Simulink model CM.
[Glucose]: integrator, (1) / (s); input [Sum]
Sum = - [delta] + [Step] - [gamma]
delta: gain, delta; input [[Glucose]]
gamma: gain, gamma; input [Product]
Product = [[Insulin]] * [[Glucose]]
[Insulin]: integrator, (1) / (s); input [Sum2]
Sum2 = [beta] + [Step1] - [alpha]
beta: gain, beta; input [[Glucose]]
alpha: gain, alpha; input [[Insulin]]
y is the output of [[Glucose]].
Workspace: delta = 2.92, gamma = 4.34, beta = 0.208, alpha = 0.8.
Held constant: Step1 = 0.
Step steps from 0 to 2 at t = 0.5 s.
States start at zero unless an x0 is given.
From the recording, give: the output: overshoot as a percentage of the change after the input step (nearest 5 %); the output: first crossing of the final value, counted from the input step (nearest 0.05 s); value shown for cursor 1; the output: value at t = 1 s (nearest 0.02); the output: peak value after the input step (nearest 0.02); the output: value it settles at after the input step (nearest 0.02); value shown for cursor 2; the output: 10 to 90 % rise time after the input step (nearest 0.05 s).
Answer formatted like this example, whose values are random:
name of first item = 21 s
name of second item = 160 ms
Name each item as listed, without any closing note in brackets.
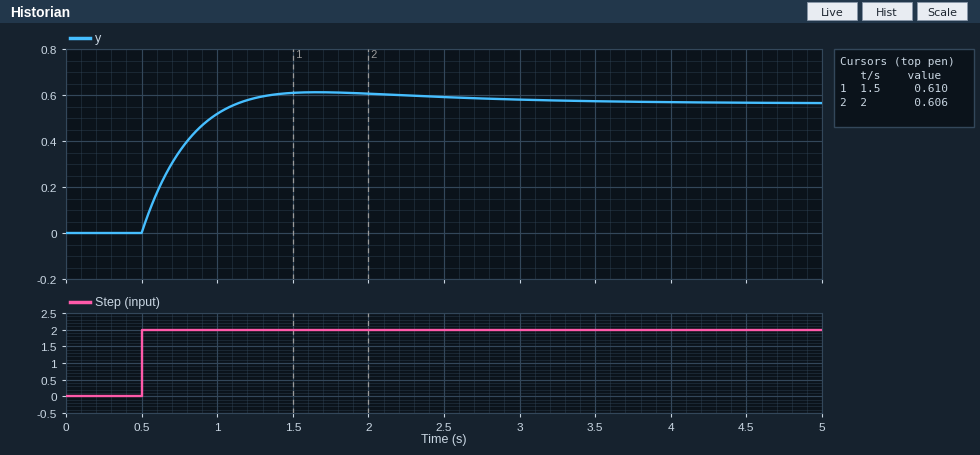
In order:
the output: overshoot as a percentage of the change after the input step = 10 %
the output: first crossing of the final value, counted from the input step = 0.65 s
value shown for cursor 1 = 0.610
the output: value at t = 1 s = 0.52
the output: peak value after the input step = 0.62
the output: value it settles at after the input step = 0.56
value shown for cursor 2 = 0.606
the output: 10 to 90 % rise time after the input step = 0.45 s
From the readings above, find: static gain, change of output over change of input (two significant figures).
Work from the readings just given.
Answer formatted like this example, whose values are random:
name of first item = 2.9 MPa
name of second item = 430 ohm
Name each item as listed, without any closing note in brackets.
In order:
static gain, change of output over change of input = 0.28
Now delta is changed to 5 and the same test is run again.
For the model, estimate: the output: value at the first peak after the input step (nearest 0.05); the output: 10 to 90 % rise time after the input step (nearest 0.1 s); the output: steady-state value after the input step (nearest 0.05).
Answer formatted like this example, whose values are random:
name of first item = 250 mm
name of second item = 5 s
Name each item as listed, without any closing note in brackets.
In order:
the output: value at the first peak after the input step = 0.40
the output: 10 to 90 % rise time after the input step = 0.3 s
the output: steady-state value after the input step = 0.35
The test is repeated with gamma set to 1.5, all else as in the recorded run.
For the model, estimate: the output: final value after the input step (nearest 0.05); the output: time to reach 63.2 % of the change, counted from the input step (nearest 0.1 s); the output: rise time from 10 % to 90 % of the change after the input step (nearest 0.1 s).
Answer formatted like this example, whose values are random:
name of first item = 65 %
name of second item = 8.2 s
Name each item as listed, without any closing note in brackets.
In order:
the output: final value after the input step = 0.65
the output: time to reach 63.2 % of the change, counted from the input step = 0.3 s
the output: rise time from 10 % to 90 % of the change after the input step = 0.6 s
